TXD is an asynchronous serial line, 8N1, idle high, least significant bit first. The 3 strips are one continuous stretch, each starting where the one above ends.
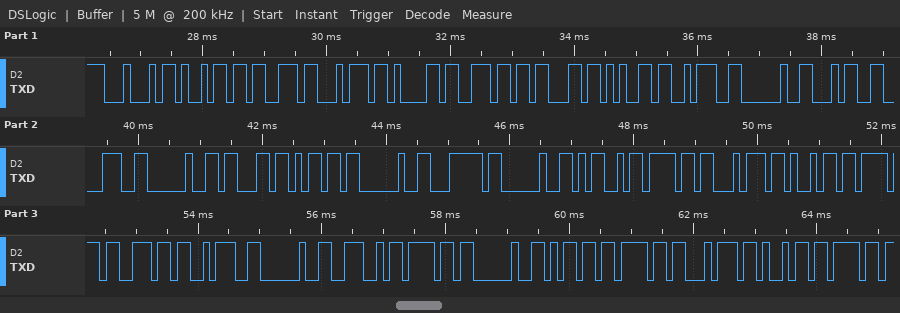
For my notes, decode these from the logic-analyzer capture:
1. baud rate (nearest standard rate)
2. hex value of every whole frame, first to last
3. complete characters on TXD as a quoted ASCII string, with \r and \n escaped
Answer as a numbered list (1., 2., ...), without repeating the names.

1. 9600 baud
2. 44 69 73 74 61 6E 63 65 3A 20 34 38 20 63 6D 20 7C 20 4D 6F 74 69 6F 6E 3A 20 4E 6F 20 6D 6F 74 69 6F
3. "Distance: 48 cm | Motion: No motio"
